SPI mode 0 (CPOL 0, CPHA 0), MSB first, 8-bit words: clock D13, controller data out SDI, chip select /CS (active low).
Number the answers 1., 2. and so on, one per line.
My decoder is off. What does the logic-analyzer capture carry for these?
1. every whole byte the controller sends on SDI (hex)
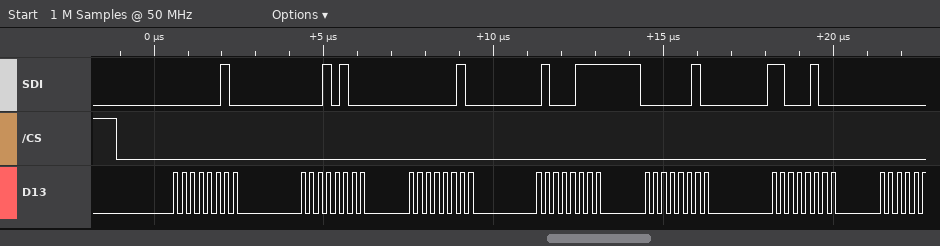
1. 02 14 02 47 02 C4
